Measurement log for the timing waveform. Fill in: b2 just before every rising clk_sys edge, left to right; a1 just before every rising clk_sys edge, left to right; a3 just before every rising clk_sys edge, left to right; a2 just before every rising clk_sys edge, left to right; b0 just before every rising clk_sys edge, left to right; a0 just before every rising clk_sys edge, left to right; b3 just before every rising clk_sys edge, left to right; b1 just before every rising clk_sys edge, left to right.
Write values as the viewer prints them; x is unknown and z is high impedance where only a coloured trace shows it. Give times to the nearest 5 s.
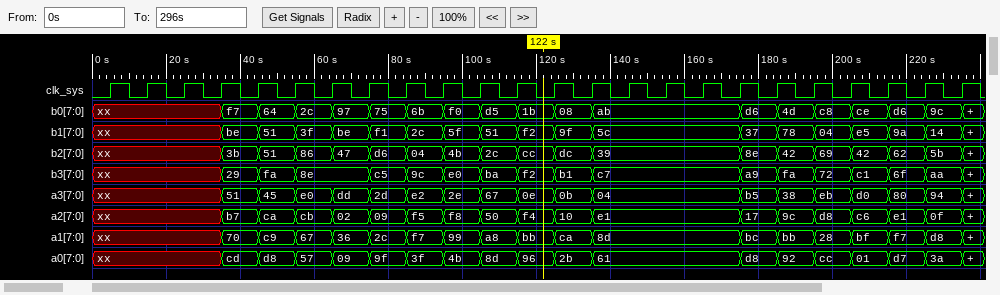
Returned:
xx, xx, xx, xx, 3b, 51, 86, 47, d6, 04, 4b, 2c, cc, dc, 39, 39, 39, 39, 8e, 42, 69, 42, 62, 5b
xx, xx, xx, xx, 70, c9, 67, 36, 2c, f7, 99, a8, bb, ca, 8d, 8d, 8d, 8d, bc, bb, 28, bf, f7, d8
xx, xx, xx, xx, 51, 45, e0, dd, 2d, e2, 2e, 67, 0e, 0b, 04, 04, 04, 04, b5, 38, eb, d0, 80, 94
xx, xx, xx, xx, b7, ca, cb, 02, 09, f5, f8, 50, f4, 10, e1, e1, e1, e1, 17, 9c, d8, c6, e1, 0f
xx, xx, xx, xx, f7, 64, 2c, 97, 75, 6b, f0, d5, 1b, 08, ab, ab, ab, ab, d6, 4d, c8, ce, d6, 9c
xx, xx, xx, xx, cd, d8, 57, 09, 9f, 3f, 4b, 8d, 96, 2b, 61, 61, 61, 61, d8, 92, cc, 01, d7, 3a
xx, xx, xx, xx, 29, fa, 8e, 8e, c5, 9c, e0, ba, f2, b1, c7, c7, c7, c7, a9, fa, 72, c1, 6f, aa
xx, xx, xx, xx, be, 51, 3f, be, f1, 2c, 5f, 51, f2, 9f, 5c, 5c, 5c, 5c, 37, 78, 04, e5, 9a, 14
